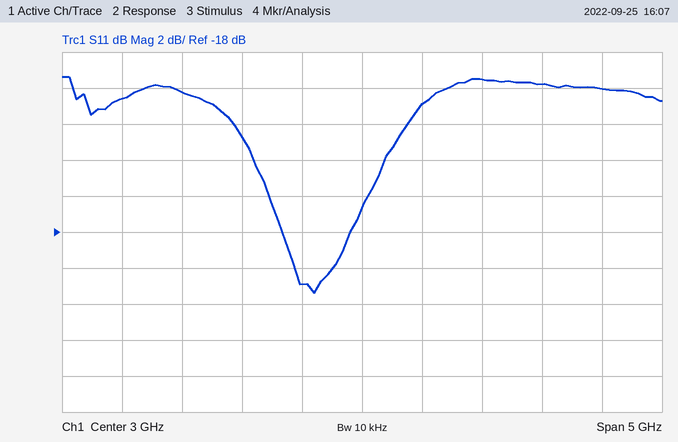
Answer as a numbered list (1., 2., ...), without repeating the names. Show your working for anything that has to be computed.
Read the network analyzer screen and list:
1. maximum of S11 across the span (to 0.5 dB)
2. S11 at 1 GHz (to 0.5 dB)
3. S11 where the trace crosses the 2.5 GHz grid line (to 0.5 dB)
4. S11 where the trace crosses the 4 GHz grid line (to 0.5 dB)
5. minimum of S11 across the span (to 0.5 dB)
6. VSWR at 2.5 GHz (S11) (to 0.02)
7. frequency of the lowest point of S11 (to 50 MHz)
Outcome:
1. -9.5 dB
2. -10.5 dB
3. -21.0 dB
4. -9.5 dB
5. -21.5 dB
6. |Γ| = 10^(-21/20) = 0.0891; VSWR = (1 + 0.0891)/(1 − 0.0891) ≈ 1.20
7. 2.60 GHz
